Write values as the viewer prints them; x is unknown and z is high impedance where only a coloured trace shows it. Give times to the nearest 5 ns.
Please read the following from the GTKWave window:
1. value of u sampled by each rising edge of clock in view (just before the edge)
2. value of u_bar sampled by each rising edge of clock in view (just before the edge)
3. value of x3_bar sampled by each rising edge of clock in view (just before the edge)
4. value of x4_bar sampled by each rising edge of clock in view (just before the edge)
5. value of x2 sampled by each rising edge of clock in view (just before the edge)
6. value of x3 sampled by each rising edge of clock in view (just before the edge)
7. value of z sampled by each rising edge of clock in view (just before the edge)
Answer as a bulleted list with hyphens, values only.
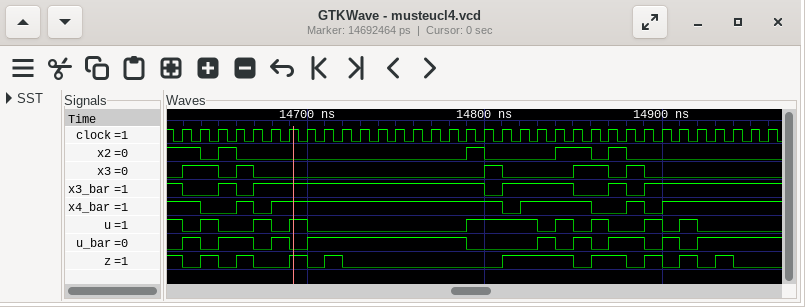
- 1 0 1 0 0 1 0 1 0 0 0 0 0 0 0 0 0 1 1 1 1 0 1 0 1 0 0 1 0 1 0 0 0 0
- 0 1 0 1 1 0 1 0 1 1 1 1 1 1 1 1 1 0 0 0 0 1 0 1 0 1 1 0 1 0 1 1 1 1
- 1 0 0 1 0 1 1 1 1 1 1 1 1 1 1 1 1 1 0 1 1 1 1 0 0 1 0 1 1 1 1 1 1 1
- 1 1 0 0 1 0 1 1 1 1 1 1 1 1 1 1 1 1 1 0 1 1 1 1 0 0 1 0 1 1 1 1 1 1
- 1 1 0 1 0 0 0 0 0 0 0 0 0 0 0 0 0 1 0 0 0 0 1 1 0 1 0 0 0 0 0 0 0 0
- 0 1 1 0 1 0 0 0 0 0 0 0 0 0 0 0 0 0 1 0 0 0 0 1 1 0 1 0 0 0 0 0 0 0
- 1 0 1 0 1 0 0 1 0 1 0 0 0 0 0 0 0 0 0 1 1 1 1 0 1 1 0 1 0 1 0 1 0 0
